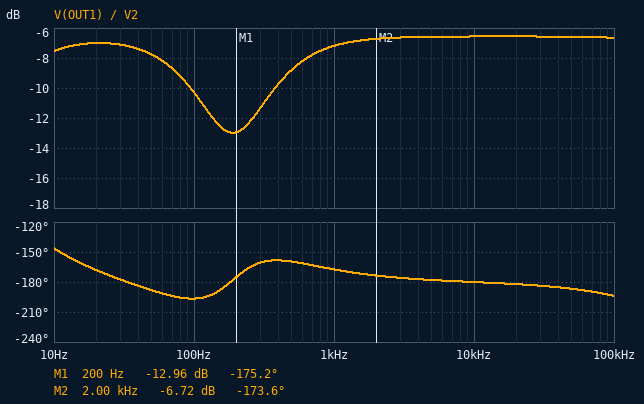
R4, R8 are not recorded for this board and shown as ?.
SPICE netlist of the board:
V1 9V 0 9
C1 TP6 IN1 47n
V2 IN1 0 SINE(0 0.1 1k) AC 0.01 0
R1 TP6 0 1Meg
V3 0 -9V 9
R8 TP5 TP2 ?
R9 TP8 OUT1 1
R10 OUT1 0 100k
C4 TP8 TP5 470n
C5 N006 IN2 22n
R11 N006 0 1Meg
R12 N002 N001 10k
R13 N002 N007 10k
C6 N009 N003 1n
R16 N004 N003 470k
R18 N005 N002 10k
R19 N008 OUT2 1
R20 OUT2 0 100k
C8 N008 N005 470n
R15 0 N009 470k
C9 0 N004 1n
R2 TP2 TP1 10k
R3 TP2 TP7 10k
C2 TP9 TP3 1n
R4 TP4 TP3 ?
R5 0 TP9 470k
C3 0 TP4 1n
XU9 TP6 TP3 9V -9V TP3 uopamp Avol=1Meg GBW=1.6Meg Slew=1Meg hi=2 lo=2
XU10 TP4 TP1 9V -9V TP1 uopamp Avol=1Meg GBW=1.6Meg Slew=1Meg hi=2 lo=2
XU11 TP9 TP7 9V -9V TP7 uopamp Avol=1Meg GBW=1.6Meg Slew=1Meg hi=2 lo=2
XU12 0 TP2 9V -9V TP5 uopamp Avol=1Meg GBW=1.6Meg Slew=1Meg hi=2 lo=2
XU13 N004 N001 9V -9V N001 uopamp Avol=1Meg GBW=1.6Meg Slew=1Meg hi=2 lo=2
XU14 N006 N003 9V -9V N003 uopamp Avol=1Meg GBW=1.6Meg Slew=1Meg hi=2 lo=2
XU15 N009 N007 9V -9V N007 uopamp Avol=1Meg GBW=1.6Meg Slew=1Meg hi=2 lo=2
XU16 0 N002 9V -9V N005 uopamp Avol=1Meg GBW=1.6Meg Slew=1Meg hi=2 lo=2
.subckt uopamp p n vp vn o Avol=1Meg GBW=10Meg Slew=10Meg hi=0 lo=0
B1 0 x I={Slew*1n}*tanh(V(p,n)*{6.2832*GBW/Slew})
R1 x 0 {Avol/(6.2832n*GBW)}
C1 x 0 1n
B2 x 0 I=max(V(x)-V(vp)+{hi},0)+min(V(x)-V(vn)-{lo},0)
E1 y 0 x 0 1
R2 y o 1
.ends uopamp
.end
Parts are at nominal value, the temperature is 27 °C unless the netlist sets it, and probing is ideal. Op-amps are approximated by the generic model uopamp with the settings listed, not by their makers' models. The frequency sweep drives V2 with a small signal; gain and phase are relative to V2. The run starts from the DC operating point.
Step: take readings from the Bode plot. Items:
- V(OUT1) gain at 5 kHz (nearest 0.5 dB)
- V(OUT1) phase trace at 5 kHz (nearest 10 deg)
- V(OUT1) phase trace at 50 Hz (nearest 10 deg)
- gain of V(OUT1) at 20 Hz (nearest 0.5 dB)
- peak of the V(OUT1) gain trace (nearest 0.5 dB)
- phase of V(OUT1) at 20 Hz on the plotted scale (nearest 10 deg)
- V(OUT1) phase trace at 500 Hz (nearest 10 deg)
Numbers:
-6.5 dB
-180 deg
-190 deg
-7.0 dB
-6.5 dB
-170 deg
-160 deg
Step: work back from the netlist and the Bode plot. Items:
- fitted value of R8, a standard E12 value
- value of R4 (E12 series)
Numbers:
4.7 kΩ
1.5 MΩ
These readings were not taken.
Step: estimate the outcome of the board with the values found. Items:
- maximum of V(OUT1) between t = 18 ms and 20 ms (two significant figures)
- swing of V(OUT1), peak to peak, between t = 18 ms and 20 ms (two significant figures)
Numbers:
44 mV
87 mV
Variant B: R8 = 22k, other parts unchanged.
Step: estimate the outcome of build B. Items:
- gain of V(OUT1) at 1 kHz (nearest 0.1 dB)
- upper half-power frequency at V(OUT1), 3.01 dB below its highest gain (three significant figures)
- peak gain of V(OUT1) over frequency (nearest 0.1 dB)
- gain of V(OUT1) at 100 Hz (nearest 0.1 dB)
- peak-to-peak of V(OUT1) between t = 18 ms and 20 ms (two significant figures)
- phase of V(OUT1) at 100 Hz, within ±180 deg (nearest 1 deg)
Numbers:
6.2 dB
279 kHz
6.8 dB
3.1 dB
410 mV
163 deg
